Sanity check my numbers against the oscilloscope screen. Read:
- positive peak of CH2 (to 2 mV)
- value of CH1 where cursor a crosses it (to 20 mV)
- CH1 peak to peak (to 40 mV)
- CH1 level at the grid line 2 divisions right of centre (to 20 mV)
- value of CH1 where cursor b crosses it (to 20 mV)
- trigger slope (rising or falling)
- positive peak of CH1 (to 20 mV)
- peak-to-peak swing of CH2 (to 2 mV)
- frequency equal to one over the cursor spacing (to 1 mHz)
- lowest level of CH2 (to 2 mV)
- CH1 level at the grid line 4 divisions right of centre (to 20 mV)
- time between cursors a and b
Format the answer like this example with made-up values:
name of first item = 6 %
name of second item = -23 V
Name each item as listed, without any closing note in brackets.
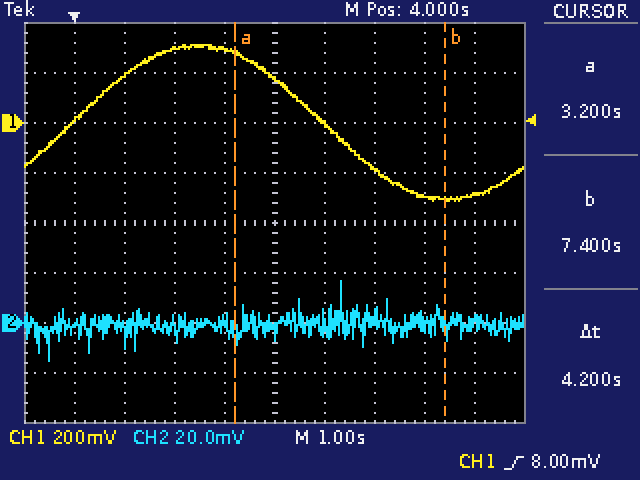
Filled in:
positive peak of CH2 = 16 mV
value of CH1 where cursor a crosses it = 280 mV
CH1 peak to peak = 640 mV
CH1 level at the grid line 2 divisions right of centre = -180 mV
value of CH1 where cursor b crosses it = -300 mV
trigger slope = rising
positive peak of CH1 = 320 mV
peak-to-peak swing of CH2 = 32 mV
frequency equal to one over the cursor spacing = 238 mHz
lowest level of CH2 = -16 mV
CH1 level at the grid line 4 divisions right of centre = -280 mV
time between cursors a and b = 4.2 s
